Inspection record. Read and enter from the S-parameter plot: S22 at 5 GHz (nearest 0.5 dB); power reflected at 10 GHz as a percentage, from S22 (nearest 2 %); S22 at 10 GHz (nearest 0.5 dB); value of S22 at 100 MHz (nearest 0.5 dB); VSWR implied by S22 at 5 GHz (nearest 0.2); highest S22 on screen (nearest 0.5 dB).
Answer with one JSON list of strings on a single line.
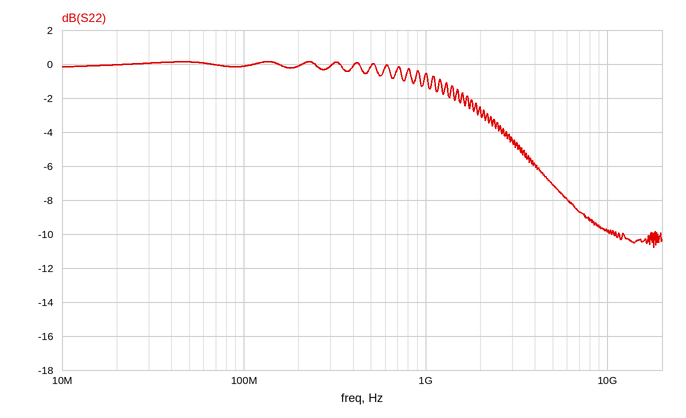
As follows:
["-7.0 dB", "10 %", "-10.0 dB", "0.0 dB", "2.6", "0.0 dB"]
